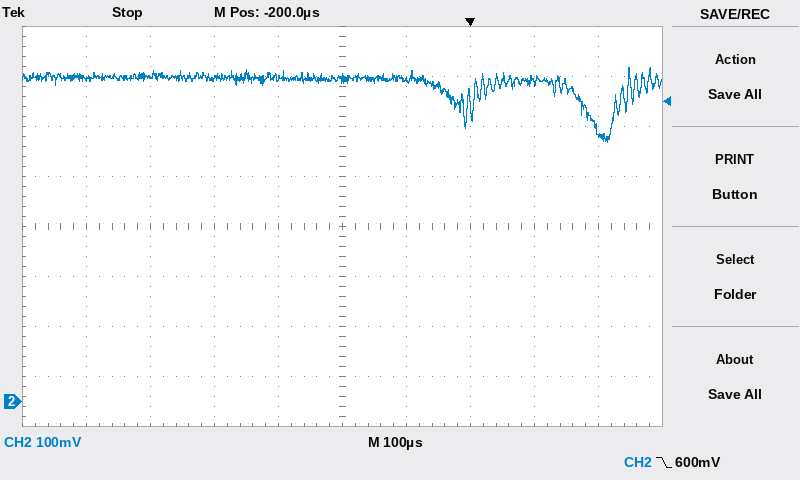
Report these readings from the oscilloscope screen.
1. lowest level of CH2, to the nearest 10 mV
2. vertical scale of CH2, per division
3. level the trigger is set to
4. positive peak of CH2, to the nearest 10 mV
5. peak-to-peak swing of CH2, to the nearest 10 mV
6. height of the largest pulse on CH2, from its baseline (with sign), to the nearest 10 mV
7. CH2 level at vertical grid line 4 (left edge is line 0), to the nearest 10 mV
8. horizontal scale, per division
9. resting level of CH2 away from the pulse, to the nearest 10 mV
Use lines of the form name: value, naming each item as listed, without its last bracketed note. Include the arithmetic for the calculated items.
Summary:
lowest level of CH2, to the nearest 10 mV: 520 mV
vertical scale of CH2, per division: 100 mV
level the trigger is set to: 600 mV
positive peak of CH2, to the nearest 10 mV: 670 mV
peak-to-peak swing of CH2, to the nearest 10 mV: 670 mV − (520 mV) = 150 mV
height of the largest pulse on CH2, from its baseline (with sign), to the nearest 10 mV: 520 mV − (650 mV) = -130 mV
CH2 level at vertical grid line 4 (left edge is line 0), to the nearest 10 mV: 650 mV
horizontal scale, per division: 100 µs
resting level of CH2 away from the pulse, to the nearest 10 mV: 650 mV
